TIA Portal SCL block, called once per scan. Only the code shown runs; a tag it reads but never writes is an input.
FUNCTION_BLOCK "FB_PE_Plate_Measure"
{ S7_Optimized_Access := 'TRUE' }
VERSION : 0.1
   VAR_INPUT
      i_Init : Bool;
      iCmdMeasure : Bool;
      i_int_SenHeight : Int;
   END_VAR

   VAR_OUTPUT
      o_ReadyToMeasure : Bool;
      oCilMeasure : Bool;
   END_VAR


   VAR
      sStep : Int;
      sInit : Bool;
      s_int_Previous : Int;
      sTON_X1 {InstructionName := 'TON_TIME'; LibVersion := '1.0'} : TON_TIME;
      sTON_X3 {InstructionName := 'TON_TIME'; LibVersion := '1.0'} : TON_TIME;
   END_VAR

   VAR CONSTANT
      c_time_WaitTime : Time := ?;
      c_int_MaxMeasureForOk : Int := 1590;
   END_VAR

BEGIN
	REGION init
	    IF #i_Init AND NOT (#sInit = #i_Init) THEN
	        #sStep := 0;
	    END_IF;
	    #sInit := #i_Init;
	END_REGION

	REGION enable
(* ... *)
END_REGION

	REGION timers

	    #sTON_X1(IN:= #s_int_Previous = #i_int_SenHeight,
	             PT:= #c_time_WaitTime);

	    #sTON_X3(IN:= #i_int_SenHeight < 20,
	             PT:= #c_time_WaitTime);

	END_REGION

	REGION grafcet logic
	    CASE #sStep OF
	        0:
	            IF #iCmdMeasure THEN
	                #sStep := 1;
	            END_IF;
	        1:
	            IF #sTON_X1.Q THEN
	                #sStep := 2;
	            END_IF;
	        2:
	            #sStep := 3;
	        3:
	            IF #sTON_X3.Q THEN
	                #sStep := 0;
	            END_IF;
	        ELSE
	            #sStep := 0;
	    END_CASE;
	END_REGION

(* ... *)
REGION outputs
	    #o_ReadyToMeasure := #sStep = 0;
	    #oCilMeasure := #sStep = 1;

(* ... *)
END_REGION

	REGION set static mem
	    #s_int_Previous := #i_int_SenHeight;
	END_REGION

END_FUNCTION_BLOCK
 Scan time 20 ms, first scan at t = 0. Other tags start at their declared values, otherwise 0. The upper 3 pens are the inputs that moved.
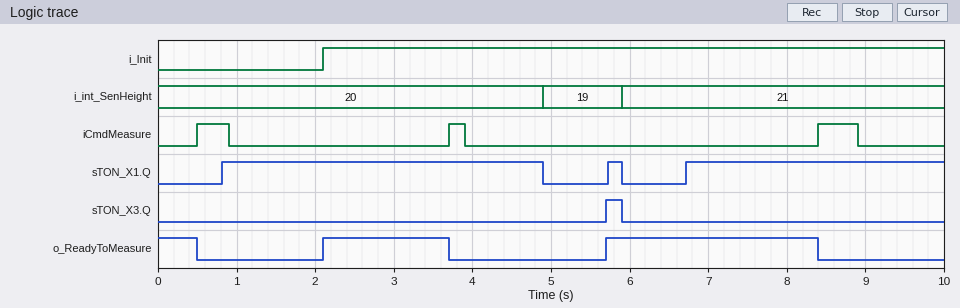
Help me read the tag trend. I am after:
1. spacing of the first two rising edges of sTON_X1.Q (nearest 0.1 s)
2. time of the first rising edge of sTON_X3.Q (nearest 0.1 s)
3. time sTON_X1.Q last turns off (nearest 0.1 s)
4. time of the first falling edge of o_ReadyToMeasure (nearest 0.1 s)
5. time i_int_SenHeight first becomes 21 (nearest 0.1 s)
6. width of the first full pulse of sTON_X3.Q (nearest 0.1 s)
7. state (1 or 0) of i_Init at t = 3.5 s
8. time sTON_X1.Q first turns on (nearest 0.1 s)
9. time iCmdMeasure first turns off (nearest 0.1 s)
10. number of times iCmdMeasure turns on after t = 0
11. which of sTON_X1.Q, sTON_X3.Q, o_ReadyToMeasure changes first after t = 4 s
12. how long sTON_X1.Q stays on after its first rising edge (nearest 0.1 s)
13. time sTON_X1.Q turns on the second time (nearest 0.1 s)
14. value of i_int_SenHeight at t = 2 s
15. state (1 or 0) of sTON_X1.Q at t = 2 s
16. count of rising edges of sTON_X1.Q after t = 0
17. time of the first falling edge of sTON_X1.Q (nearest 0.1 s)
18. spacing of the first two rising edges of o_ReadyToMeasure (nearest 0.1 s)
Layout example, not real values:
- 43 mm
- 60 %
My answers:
- 4.9 s
- 5.7 s
- 5.9 s
- 0.5 s
- 5.9 s
- 0.2 s
- 1
- 0.8 s
- 0.9 s
- 3
- sTON_X1.Q
- 4.1 s
- 5.7 s
- 20
- 1
- 3
- 4.9 s
- 3.6 s
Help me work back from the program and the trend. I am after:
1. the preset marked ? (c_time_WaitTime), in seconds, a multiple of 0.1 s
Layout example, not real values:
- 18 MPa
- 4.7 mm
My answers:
- 0.8 s
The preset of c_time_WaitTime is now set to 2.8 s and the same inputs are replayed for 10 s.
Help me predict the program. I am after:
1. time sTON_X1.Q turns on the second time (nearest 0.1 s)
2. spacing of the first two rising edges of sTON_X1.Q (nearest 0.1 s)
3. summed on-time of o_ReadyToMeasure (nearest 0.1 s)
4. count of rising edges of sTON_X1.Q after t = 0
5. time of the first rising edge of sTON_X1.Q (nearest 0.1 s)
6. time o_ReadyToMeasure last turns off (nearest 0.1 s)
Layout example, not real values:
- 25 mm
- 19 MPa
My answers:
- 8.7 s
- 5.9 s
- 2.1 s
- 2
- 2.8 s
- 3.7 s
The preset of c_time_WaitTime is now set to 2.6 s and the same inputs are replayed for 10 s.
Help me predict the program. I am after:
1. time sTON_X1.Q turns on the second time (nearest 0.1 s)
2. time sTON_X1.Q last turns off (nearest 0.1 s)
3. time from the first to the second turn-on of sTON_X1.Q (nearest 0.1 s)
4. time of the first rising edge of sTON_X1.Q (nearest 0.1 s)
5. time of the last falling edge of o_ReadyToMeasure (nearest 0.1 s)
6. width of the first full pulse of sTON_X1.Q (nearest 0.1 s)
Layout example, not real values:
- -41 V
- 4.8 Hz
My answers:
- 8.5 s
- 4.9 s
- 5.9 s
- 2.6 s
- 3.7 s
- 2.3 s
